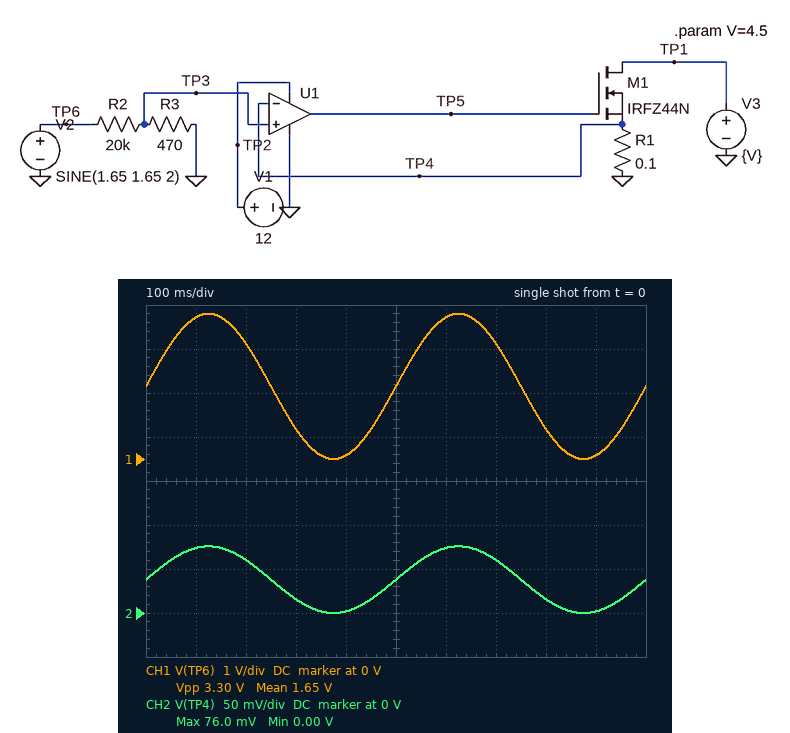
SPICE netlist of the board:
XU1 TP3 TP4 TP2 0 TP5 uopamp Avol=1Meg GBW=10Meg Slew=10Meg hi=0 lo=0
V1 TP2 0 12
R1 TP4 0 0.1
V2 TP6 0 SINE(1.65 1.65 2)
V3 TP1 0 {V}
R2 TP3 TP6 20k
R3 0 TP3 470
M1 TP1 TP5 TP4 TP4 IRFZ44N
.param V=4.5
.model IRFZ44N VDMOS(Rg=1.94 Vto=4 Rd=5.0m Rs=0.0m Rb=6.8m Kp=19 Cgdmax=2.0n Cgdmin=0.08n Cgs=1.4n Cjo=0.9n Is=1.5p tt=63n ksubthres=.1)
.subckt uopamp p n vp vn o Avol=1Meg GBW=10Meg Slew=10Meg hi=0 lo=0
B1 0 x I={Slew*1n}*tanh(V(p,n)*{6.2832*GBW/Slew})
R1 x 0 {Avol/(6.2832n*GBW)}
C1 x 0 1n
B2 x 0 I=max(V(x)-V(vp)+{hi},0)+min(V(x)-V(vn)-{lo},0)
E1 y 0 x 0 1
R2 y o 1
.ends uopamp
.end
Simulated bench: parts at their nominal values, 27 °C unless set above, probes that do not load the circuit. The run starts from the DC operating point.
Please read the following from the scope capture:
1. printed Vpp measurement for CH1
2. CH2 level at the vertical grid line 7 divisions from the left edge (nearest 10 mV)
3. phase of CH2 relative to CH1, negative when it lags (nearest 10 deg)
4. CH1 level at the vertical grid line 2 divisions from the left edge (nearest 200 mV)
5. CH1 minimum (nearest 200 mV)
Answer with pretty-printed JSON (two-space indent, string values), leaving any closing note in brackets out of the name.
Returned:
{
  "printed Vpp measurement for CH1": "3.30 V",
  "CH2 level at the vertical grid line 7 divisions from the left edge": "60 mV",
  "phase of CH2 relative to CH1, negative when it lags": "0 deg",
  "CH1 level at the vertical grid line 2 divisions from the left edge": "2.6 V",
  "CH1 minimum": "0 V"
}
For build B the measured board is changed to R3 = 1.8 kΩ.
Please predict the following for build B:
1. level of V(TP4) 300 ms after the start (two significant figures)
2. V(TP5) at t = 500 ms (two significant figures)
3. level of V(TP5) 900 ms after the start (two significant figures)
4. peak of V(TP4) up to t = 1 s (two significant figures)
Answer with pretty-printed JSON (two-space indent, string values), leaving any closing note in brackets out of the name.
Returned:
{
  "level of V(TP4) 300 ms after the start": "56 mV",
  "V(TP5) at t = 500 ms": "4.5 V",
  "level of V(TP5) 900 ms after the start": "4.0 V",
  "peak of V(TP4) up to t = 1 s": "270 mV"
}
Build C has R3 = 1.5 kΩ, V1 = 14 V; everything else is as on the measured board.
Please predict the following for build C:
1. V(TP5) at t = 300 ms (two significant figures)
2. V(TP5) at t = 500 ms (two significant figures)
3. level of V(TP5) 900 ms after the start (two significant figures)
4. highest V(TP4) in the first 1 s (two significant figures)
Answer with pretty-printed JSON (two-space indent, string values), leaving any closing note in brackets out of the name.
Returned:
{
  "V(TP5) at t = 300 ms": "4.3 V",
  "V(TP5) at t = 500 ms": "4.5 V",
  "level of V(TP5) 900 ms after the start": "4.0 V",
  "highest V(TP4) in the first 1 s": "230 mV"
}
